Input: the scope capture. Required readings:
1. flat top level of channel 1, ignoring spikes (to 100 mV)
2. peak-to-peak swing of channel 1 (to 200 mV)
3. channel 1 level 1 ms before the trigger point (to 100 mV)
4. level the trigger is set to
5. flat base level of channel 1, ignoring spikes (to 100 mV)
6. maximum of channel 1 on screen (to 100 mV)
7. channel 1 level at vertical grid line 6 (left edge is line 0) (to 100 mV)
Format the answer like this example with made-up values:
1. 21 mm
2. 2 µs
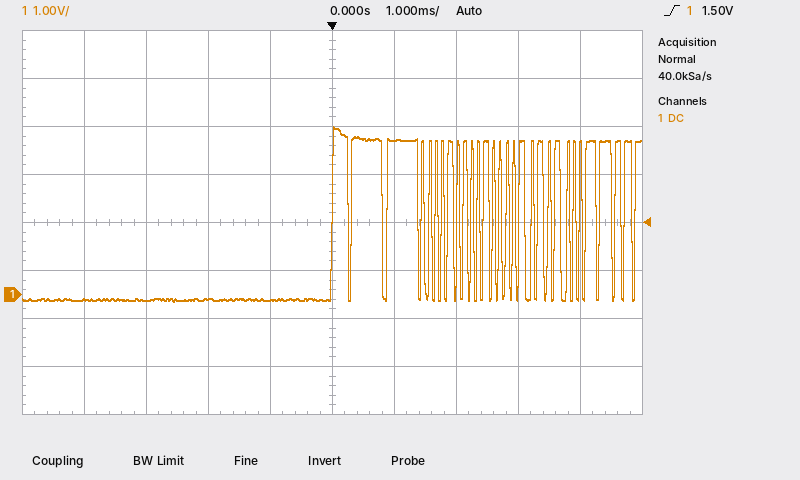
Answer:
1. 3.2 V
2. 3.6 V
3. -100 mV
4. 1.50 V
5. -100 mV
6. 3.5 V
7. 3.2 V
